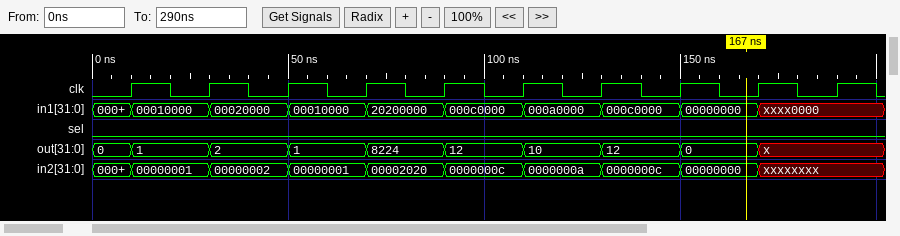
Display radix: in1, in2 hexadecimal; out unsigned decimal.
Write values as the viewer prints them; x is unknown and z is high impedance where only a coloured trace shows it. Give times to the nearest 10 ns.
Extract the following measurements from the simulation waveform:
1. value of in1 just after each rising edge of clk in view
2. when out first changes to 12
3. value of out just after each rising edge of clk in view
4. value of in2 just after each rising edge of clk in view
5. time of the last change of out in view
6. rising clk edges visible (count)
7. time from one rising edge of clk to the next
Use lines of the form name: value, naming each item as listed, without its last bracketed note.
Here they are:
value of in1 just after each rising edge of clk in view: 00010000, 00020000, 00010000, 20200000, 000c0000, 000a0000, 000c0000, 00000000, xxxx0000, xxxx0000
when out first changes to 12: 90 ns
value of out just after each rising edge of clk in view: 1, 2, 1, 8224, 12, 10, 12, 0, x, x
value of in2 just after each rising edge of clk in view: 00000001, 00000002, 00000001, 00002020, 0000000c, 0000000a, 0000000c, 00000000, xxxxxxxx, xxxxxxxx
time of the last change of out in view: 170 ns
rising clk edges visible: 10
time from one rising edge of clk to the next: 20 ns
